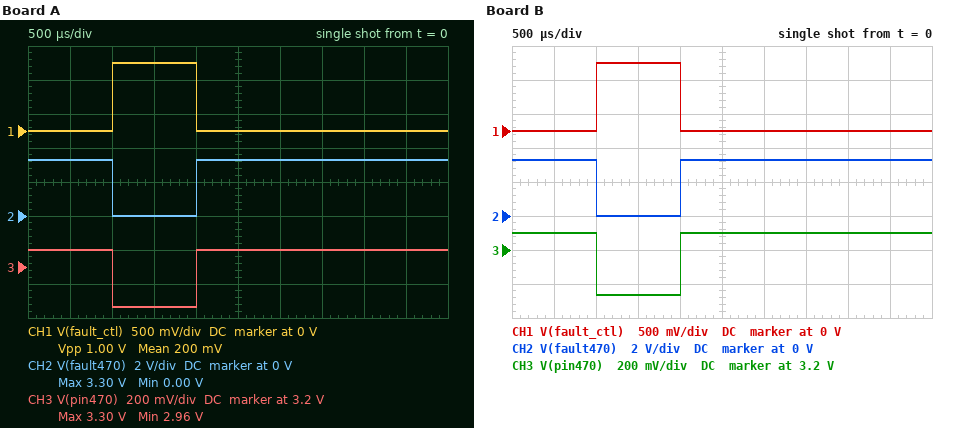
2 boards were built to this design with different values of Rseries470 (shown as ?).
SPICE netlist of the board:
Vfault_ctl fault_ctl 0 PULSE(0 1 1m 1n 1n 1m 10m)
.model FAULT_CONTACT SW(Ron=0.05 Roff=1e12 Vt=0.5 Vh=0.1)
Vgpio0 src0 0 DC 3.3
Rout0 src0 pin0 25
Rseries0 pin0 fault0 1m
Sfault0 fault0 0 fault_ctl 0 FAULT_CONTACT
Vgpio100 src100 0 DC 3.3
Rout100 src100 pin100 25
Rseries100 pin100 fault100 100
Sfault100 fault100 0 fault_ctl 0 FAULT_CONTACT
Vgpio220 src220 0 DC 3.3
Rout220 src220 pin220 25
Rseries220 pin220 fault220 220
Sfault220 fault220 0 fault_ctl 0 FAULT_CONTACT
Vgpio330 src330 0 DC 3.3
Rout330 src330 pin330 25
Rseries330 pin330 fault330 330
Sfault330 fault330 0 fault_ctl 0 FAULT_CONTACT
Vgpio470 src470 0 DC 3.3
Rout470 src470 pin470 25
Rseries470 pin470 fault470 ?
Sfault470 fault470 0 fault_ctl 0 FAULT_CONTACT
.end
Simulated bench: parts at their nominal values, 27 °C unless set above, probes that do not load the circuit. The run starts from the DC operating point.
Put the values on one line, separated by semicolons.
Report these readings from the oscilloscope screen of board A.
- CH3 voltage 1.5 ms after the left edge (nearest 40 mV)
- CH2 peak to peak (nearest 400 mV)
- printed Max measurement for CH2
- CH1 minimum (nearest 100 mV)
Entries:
2.96 V; 3.2 V; 3.30 V; 0 V
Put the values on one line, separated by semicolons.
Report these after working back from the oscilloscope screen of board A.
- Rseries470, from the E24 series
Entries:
220 Ω
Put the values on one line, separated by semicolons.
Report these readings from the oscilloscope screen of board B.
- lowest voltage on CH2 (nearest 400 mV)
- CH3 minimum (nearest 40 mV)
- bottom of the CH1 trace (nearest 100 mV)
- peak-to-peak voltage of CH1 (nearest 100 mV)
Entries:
0 V; 2.92 V; 0 V; 1.0 V
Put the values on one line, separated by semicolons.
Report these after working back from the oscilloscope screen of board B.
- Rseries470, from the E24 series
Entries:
200 Ω
